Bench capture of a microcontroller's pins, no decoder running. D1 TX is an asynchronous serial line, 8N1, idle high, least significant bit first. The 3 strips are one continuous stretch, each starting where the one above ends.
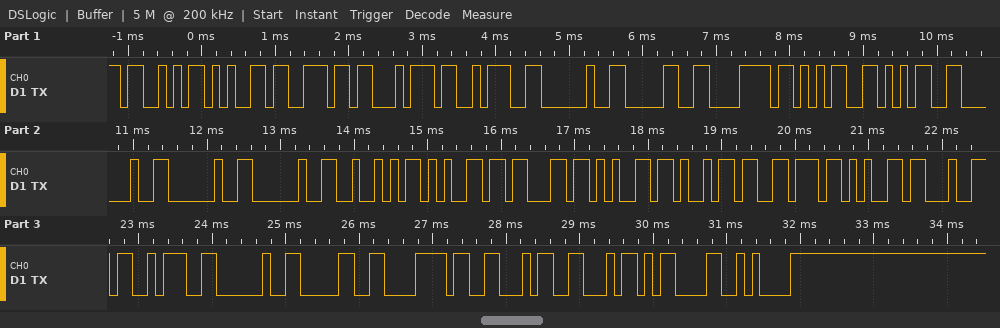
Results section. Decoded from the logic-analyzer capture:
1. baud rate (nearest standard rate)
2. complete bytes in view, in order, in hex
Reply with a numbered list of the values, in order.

1. 9600 baud
2. 53 65 6E 74 3A 20 30 78 35 35 20 20 20 52 65 63 65 69 76 65 64 3A 20 30 78 46 46 0D 0A
